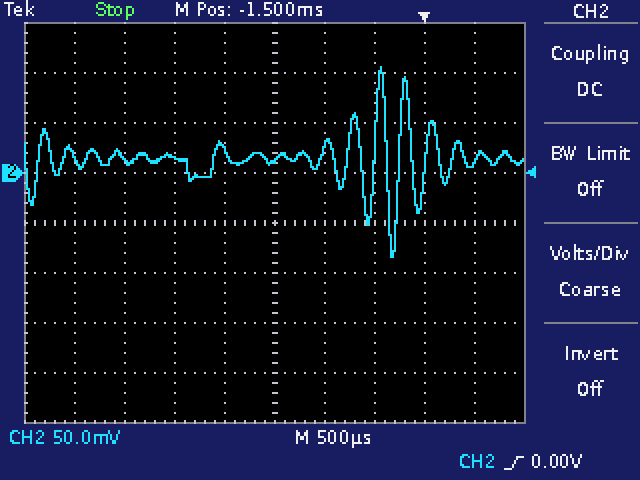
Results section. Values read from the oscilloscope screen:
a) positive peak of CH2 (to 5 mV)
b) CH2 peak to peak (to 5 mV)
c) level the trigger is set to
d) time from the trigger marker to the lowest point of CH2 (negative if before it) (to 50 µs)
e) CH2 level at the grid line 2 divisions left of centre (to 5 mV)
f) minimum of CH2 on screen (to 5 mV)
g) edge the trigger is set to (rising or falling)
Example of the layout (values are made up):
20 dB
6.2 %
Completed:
105 mV
190 mV
0.00 V
-300 µs
15 mV
-85 mV
rising
